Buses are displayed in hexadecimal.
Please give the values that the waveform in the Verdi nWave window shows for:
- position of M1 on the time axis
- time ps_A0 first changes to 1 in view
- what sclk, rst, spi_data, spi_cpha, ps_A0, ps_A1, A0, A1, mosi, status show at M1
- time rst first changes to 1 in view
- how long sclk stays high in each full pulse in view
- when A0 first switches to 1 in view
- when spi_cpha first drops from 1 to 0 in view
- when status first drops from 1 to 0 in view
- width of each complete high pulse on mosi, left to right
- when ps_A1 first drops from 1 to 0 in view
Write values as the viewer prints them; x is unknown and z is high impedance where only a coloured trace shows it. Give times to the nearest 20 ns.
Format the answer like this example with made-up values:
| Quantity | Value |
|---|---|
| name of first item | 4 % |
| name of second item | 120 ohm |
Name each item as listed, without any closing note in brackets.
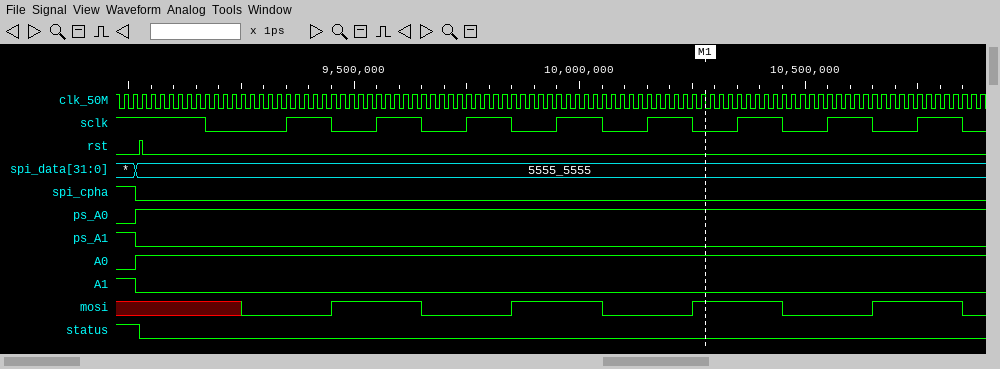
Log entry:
| Quantity | Value |
|---|---|
| position of M1 on the time axis | 10280 ns |
| time ps_A0 first changes to 1 in view | 9020 ns |
| what sclk, rst, spi_data, spi_cpha, ps_A0, ps_A1, A0, A1, mosi, status show at M1 | sclk=0, rst=0, spi_data=5555_5555, spi_cpha=0, ps_A0=1, ps_A1=0, A0=1, A1=0, mosi=1, status=0 |
| time rst first changes to 1 in view | 9020 ns |
| how long sclk stays high in each full pulse in view | 100 ns, 100 ns, 100 ns, 100 ns, 100 ns, 100 ns, 100 ns, 100 ns |
| when A0 first switches to 1 in view | 9020 ns |
| when spi_cpha first drops from 1 to 0 in view | 9020 ns |
| when status first drops from 1 to 0 in view | 9020 ns |
| width of each complete high pulse on mosi, left to right | 200 ns, 200 ns, 200 ns, 200 ns |
| when ps_A1 first drops from 1 to 0 in view | 9020 ns |
